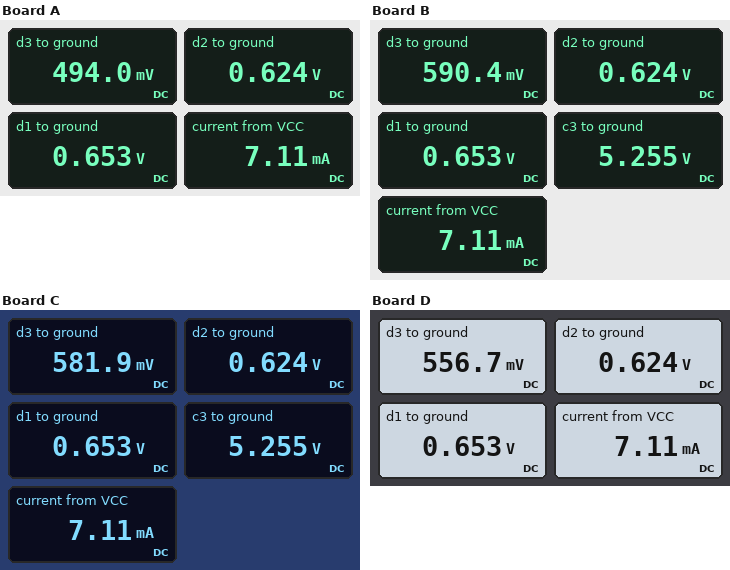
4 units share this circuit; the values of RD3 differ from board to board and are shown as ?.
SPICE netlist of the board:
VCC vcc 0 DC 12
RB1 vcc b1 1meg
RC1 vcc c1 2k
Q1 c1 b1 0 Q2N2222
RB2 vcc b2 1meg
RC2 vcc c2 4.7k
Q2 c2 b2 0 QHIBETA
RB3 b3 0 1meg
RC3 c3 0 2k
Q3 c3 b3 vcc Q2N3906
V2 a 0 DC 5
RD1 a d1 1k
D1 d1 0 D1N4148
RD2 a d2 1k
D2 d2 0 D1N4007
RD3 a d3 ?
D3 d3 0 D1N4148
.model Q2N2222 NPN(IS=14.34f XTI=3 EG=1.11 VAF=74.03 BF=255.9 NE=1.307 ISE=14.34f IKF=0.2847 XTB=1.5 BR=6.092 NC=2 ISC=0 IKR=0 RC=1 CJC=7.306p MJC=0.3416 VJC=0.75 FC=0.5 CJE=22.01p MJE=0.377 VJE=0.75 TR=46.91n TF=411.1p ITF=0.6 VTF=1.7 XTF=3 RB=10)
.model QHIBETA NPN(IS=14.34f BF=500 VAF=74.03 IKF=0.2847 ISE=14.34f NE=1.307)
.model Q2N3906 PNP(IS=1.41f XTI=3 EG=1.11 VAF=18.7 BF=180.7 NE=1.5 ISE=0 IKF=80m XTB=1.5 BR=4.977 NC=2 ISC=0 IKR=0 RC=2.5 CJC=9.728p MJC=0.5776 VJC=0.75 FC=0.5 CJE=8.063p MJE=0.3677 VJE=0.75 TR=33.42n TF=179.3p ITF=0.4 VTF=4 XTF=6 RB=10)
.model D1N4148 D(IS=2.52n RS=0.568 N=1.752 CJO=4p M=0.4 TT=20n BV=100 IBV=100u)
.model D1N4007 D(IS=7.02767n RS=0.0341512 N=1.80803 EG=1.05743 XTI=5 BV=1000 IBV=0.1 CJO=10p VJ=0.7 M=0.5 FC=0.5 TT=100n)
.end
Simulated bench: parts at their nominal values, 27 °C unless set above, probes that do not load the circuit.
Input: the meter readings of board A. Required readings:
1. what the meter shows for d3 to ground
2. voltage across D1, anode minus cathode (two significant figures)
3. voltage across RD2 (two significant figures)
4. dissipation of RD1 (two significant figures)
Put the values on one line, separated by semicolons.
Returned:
494.0 mV; 650 mV; 4.4 V; 19 mW
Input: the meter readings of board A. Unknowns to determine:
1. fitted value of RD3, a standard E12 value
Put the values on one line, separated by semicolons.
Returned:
33 kΩ
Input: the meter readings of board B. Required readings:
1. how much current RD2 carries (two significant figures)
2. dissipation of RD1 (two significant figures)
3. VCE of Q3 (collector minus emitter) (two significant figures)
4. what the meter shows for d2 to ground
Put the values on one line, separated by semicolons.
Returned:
4.4 mA; 19 mW; -6.7 V; 0.624 V
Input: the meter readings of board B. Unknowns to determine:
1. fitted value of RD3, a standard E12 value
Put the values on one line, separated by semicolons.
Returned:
3.9 kΩ
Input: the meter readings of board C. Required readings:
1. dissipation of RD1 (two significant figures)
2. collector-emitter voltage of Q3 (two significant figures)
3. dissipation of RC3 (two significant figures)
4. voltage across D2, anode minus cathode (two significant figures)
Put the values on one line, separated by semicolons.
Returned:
19 mW; -6.7 V; 14 mW; 620 mV
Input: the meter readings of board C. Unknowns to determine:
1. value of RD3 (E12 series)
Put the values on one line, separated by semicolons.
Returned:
4.7 kΩ
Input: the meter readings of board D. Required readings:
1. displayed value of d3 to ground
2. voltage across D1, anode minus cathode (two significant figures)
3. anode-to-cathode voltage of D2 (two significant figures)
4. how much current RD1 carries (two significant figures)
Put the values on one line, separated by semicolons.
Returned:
556.7 mV; 650 mV; 620 mV; 4.3 mA
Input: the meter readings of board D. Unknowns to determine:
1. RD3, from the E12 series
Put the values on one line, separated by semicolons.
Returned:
8.2 kΩ
